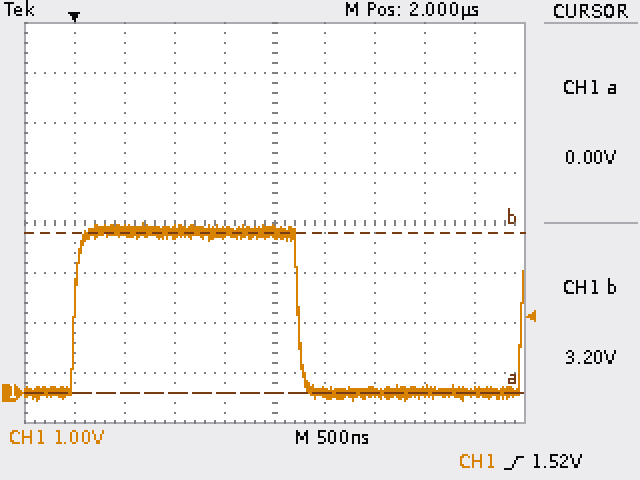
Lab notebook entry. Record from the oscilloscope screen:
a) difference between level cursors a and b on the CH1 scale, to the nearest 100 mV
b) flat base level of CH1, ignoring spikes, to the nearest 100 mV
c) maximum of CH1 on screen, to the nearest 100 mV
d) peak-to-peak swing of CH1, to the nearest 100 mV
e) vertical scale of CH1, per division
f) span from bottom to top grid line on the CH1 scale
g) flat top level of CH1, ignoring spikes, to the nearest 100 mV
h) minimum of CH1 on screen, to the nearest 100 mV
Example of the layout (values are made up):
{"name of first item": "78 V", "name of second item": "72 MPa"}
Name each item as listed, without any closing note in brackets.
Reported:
{"difference between level cursors a and b on the CH1 scale, to the nearest 100 mV": "3.2 V", "flat base level of CH1, ignoring spikes, to the nearest 100 mV": "0.0 V", "maximum of CH1 on screen, to the nearest 100 mV": "3.4 V", "peak-to-peak swing of CH1, to the nearest 100 mV": "3.6 V", "vertical scale of CH1, per division": "1 V", "span from bottom to top grid line on the CH1 scale": "8 V", "flat top level of CH1, ignoring spikes, to the nearest 100 mV": "3.2 V", "minimum of CH1 on screen, to the nearest 100 mV": "-200 mV"}
